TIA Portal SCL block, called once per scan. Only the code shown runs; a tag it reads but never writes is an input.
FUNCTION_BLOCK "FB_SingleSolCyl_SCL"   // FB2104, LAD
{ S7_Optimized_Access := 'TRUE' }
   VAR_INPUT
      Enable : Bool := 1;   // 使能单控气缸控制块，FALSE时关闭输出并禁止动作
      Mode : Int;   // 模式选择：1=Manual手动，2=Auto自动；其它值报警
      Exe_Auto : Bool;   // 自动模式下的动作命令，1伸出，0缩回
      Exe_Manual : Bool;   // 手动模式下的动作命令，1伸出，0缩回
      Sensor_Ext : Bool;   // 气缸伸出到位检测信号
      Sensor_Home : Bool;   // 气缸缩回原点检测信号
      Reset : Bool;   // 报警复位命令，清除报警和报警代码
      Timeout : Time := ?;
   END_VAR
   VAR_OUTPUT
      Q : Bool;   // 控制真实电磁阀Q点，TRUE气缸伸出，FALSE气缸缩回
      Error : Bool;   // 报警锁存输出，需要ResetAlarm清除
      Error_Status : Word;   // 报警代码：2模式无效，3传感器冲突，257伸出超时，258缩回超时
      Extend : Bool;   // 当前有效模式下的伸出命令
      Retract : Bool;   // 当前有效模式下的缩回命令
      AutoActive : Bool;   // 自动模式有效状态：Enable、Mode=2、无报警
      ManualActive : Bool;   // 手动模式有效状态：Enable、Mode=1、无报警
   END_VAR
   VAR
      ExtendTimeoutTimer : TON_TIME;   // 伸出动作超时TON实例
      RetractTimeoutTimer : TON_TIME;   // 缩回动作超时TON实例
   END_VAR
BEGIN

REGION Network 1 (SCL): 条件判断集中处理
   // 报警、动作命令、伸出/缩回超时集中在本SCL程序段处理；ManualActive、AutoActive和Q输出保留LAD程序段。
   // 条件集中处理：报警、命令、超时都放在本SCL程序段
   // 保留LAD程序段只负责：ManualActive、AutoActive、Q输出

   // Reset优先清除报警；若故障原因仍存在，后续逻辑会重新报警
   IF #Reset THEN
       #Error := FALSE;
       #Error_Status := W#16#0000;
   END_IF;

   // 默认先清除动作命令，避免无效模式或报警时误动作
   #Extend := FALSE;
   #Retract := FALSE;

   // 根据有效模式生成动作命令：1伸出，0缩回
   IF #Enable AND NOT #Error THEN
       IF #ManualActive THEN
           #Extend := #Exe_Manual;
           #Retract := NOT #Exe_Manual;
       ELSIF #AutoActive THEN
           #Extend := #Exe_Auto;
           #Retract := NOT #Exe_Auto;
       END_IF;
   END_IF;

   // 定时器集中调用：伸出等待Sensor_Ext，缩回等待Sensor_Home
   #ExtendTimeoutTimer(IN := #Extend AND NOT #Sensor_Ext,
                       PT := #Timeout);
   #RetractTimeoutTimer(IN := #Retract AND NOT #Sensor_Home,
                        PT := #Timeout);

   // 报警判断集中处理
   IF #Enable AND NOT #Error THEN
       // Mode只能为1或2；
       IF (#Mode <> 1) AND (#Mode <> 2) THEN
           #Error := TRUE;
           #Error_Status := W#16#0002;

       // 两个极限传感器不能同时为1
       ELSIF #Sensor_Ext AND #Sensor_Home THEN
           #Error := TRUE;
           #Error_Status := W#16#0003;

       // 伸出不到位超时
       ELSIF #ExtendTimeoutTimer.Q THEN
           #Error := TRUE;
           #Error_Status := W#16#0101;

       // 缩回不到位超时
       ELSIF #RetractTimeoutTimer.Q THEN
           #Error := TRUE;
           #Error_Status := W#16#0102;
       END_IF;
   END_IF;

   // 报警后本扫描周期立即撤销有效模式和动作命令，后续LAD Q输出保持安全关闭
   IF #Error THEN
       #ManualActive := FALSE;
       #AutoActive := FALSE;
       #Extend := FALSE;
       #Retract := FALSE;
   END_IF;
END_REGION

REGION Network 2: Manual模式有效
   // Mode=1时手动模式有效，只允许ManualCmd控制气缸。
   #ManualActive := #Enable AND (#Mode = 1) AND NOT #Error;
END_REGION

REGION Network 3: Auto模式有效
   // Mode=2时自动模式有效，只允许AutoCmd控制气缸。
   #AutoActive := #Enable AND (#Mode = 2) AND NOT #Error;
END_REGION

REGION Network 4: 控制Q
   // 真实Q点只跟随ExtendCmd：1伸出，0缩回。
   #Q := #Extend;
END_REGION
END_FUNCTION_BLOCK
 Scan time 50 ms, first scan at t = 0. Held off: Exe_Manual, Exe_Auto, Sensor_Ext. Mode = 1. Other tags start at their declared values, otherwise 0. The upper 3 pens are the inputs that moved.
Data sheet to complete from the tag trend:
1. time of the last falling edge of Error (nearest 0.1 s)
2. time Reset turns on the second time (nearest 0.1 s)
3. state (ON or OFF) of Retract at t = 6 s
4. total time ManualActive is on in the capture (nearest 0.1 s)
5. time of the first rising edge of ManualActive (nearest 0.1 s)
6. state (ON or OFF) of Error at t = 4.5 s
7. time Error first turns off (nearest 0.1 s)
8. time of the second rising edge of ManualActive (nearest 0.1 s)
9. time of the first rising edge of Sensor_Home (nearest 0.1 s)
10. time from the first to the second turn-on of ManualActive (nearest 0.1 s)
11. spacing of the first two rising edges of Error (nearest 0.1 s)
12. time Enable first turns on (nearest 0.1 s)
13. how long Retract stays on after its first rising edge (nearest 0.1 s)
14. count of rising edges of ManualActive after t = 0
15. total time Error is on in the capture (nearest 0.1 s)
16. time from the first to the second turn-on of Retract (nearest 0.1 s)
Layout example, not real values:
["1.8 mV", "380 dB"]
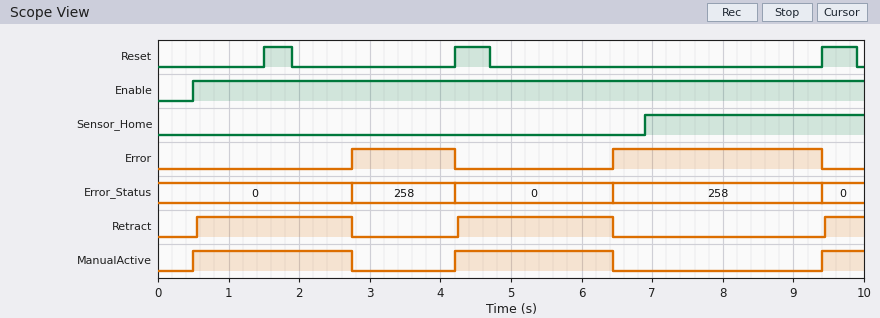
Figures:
["9.4 s", "4.2 s", "ON", "5.1 s", "0.5 s", "OFF", "4.2 s", "4.2 s", "6.9 s", "3.7 s", "3.7 s", "0.5 s", "2.2 s", "3", "4.4 s", "3.7 s"]
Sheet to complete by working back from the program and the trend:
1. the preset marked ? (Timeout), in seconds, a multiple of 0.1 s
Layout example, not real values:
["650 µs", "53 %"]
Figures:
["2.2 s"]
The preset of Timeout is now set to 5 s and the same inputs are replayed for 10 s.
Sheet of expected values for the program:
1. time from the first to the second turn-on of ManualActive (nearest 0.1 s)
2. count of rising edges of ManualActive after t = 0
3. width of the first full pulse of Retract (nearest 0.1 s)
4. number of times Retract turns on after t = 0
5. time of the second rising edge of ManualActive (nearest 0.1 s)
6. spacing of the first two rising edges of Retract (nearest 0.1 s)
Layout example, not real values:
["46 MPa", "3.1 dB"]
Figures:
["8.9 s", "2", "5.0 s", "2", "9.4 s", "8.9 s"]
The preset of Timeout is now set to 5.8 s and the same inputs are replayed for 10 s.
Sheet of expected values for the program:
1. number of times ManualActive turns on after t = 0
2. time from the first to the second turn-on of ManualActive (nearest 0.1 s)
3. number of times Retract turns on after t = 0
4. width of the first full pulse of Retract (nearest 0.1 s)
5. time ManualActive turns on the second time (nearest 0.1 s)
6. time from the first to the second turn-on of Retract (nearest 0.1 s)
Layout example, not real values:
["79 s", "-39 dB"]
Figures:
["2", "8.9 s", "2", "5.8 s", "9.4 s", "8.9 s"]
